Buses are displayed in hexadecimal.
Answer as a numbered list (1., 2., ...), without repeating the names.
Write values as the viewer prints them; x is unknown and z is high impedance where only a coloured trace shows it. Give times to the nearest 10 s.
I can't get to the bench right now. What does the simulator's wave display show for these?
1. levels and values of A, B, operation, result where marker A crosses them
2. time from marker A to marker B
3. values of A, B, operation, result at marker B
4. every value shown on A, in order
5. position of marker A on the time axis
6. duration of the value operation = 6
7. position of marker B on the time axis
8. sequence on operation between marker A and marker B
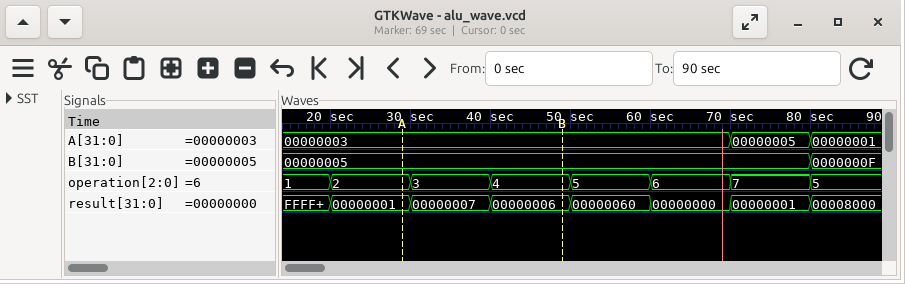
1. A=00000003, B=00000005, operation=2, result=00000001
2. 20 s
3. A=00000003, B=00000005, operation=4, result=00000006
4. 00000003, 00000005, 00000001
5. 30 s
6. 10 s
7. 50 s
8. 2, 3, 4
